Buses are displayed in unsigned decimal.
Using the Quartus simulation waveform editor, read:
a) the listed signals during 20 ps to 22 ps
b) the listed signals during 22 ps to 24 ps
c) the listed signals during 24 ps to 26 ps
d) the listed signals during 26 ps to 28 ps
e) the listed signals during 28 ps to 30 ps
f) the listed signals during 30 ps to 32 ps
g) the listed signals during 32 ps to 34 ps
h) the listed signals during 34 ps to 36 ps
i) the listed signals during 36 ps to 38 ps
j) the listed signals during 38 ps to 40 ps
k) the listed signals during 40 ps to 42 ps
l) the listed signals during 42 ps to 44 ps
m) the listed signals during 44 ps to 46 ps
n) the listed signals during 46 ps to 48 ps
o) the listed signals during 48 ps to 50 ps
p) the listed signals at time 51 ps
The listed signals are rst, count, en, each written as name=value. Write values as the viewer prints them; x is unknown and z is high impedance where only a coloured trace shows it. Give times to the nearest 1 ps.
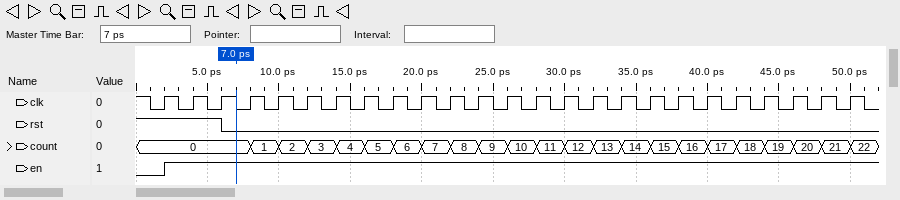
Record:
rst=0, count=7, en=1
rst=0, count=8, en=1
rst=0, count=9, en=1
rst=0, count=10, en=1
rst=0, count=11, en=1
rst=0, count=12, en=1
rst=0, count=13, en=1
rst=0, count=14, en=1
rst=0, count=15, en=1
rst=0, count=16, en=1
rst=0, count=17, en=1
rst=0, count=18, en=1
rst=0, count=19, en=1
rst=0, count=20, en=1
rst=0, count=21, en=1
rst=0, count=22, en=1
